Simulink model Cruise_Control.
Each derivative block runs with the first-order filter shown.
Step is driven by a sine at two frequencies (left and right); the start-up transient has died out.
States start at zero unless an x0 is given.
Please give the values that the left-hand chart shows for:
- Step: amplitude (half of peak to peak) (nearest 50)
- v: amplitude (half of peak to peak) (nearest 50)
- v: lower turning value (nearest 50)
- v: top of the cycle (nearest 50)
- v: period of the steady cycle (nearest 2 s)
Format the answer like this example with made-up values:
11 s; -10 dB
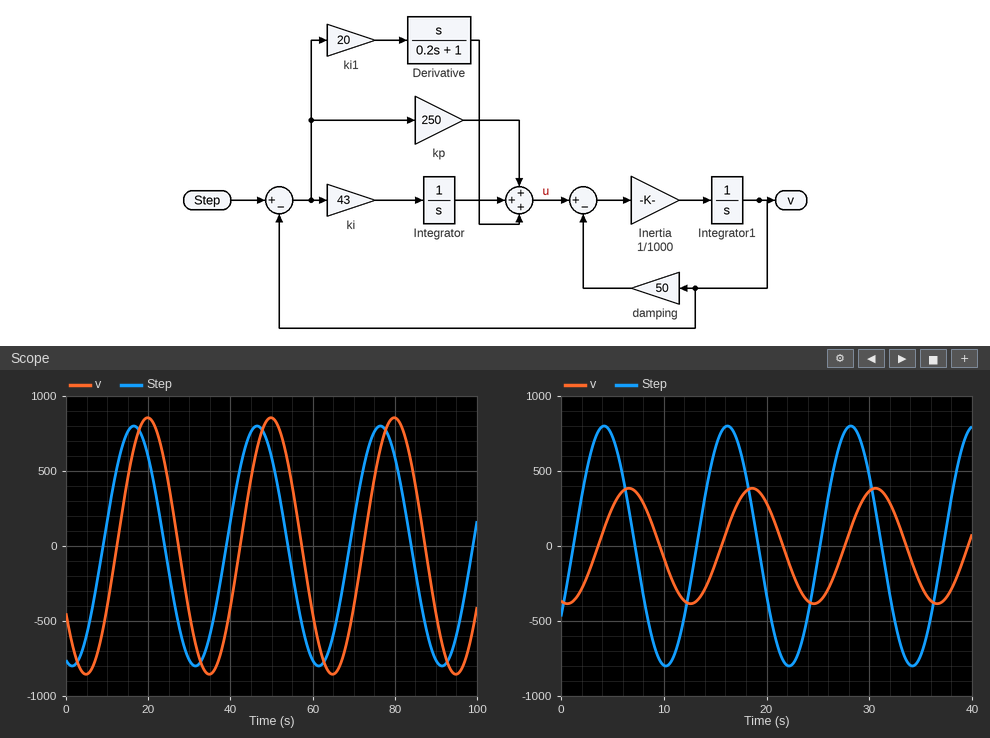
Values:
800; 850; -850; 850; 30 s
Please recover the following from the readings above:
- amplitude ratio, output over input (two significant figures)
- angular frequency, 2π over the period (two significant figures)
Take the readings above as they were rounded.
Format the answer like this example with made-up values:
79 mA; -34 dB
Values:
1.1; 0.21 rad/s
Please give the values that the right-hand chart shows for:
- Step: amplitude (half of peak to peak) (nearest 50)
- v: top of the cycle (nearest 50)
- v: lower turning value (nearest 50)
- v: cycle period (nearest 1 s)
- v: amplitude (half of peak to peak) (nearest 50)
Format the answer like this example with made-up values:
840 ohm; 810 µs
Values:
800; 400; -400; 12 s; 400
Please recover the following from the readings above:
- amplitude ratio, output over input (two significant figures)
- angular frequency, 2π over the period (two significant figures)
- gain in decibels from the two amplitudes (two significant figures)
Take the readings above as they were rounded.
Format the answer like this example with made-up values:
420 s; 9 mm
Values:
0.50; 0.52 rad/s; -6.0 dB
